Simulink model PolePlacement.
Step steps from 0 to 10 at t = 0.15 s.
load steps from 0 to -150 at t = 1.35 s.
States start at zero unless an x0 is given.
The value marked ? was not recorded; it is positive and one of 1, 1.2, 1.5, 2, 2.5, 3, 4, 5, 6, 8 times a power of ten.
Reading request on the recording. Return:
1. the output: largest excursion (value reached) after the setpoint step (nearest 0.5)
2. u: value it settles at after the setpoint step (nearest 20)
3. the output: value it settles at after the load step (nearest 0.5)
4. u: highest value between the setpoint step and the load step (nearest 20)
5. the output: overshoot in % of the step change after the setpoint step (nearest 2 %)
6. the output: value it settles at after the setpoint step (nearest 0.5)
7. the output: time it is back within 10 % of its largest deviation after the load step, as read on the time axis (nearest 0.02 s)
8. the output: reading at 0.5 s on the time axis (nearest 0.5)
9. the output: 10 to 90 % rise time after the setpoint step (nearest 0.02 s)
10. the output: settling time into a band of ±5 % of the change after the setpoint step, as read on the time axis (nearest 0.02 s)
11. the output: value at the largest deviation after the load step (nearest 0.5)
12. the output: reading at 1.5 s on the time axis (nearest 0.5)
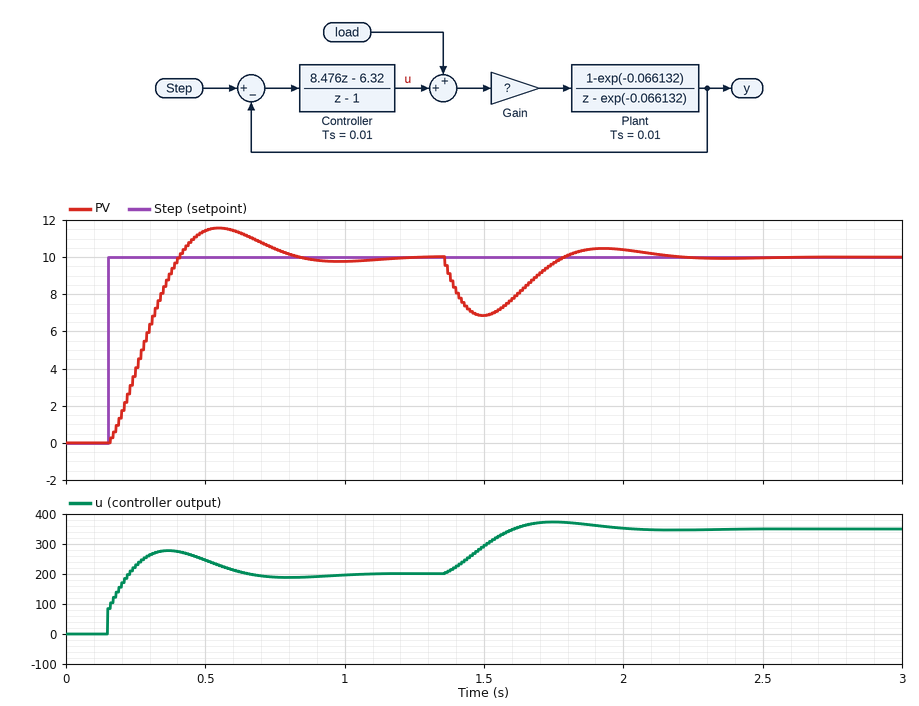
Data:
11.5
200
10.0
280
16 %
10.0
2.04 s
11.5
0.18 s
0.74 s
7.0
7.0
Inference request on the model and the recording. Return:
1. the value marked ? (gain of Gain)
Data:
0.05
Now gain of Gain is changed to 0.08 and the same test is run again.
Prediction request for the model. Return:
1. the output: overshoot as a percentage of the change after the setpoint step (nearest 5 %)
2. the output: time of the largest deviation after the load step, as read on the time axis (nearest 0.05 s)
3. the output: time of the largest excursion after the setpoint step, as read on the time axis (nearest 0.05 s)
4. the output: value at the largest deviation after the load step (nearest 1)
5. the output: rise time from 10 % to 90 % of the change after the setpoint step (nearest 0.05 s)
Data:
20 %
1.45 s
0.45 s
6
0.15 s
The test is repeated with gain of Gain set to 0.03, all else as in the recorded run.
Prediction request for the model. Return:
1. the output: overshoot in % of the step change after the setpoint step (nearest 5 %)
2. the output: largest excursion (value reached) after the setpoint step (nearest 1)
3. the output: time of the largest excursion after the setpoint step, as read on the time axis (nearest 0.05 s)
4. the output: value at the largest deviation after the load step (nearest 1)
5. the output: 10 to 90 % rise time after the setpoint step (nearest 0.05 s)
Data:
10 %
11
0.70 s
8
0.30 s
